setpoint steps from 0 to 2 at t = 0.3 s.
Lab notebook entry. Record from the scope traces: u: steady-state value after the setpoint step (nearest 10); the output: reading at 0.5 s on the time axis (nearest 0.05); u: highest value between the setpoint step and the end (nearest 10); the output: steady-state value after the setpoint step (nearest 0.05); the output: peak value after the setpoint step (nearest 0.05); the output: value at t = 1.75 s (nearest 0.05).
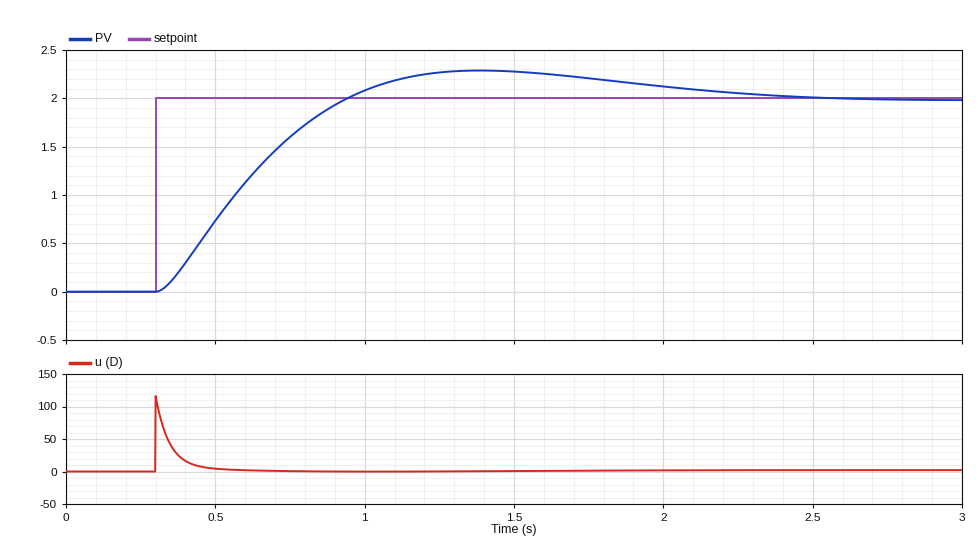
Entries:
0
0.75
120
2.00
2.30
2.20
